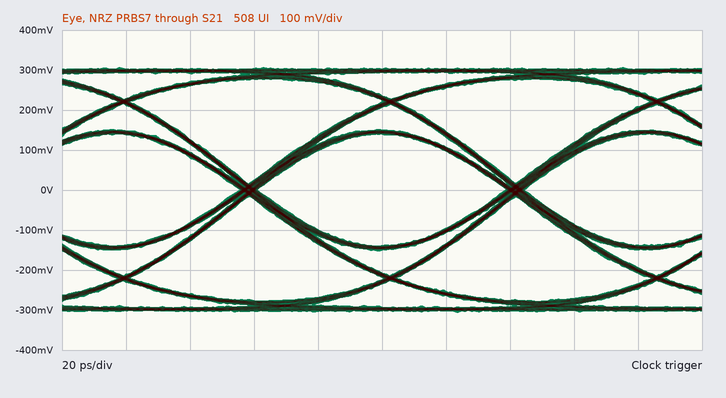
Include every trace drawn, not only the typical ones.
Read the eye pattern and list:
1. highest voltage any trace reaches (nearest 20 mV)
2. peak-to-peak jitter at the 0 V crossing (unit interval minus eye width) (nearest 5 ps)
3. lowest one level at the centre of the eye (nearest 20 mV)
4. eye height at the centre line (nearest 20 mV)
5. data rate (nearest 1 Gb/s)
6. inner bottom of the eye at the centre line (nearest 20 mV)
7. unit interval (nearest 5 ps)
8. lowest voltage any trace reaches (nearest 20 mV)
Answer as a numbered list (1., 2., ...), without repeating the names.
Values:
1. 300 mV
2. 5 ps
3. 140 mV
4. 280 mV
5. 12 Gb/s
6. -140 mV
7. 85 ps
8. -300 mV
